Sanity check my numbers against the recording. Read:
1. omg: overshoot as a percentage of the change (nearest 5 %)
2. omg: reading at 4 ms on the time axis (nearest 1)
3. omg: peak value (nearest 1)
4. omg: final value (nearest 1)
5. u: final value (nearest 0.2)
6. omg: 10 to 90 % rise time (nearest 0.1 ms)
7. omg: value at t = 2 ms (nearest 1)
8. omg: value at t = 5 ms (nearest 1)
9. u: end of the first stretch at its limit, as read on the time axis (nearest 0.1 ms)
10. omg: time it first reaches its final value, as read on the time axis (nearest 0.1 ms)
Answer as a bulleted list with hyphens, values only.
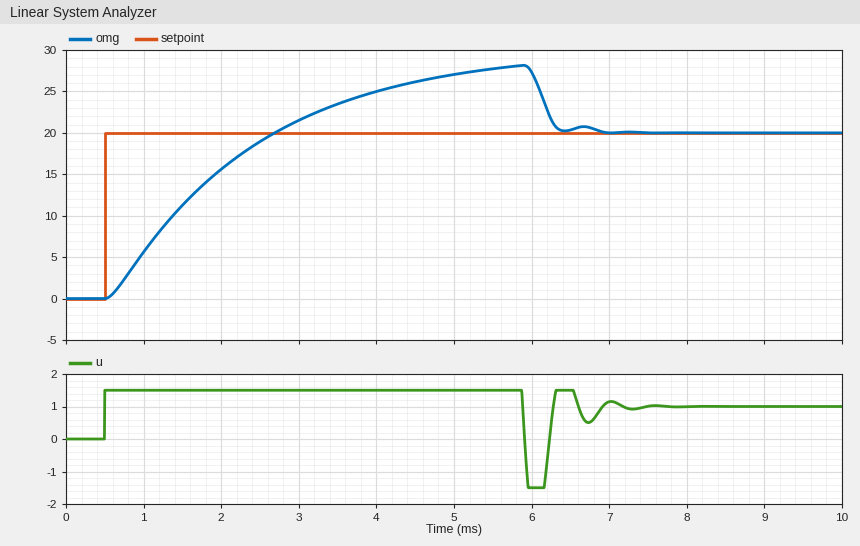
- 40 %
- 25
- 28
- 20
- 1.0
- 1.6 ms
- 16
- 27
- 5.9 ms
- 2.7 ms
